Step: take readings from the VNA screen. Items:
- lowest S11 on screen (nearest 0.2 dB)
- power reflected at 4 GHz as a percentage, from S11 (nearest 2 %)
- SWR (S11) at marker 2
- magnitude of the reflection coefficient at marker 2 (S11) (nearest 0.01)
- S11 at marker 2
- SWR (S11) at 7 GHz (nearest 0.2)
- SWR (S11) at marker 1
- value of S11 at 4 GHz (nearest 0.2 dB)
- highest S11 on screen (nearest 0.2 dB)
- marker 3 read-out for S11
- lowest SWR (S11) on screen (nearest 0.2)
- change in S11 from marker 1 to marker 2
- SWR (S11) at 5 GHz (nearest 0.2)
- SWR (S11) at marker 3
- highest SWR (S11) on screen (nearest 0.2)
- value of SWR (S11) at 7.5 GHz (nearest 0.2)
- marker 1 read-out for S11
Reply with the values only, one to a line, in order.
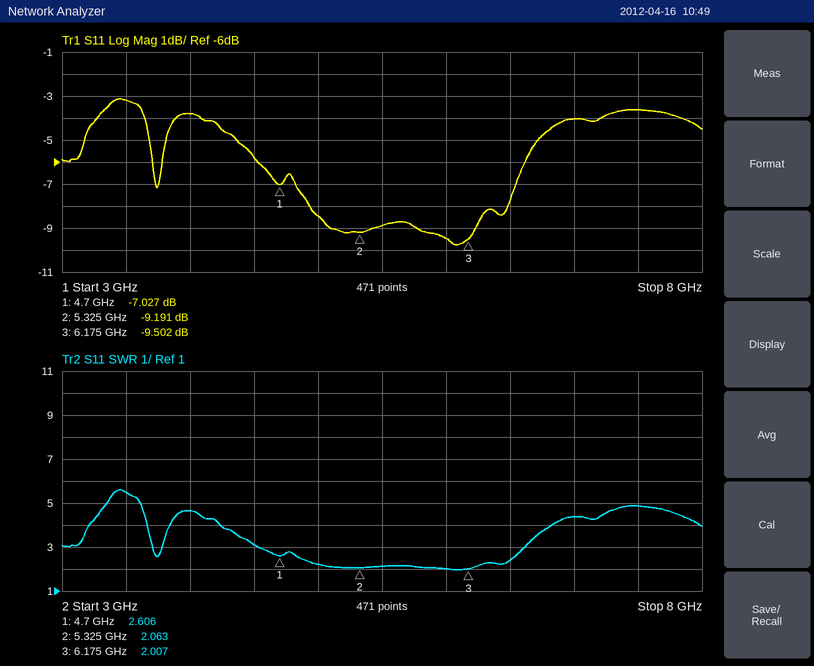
-9.8 dB
42 %
2.063
0.35
-9.191 dB
4.4
2.606
-3.8 dB
-3.2 dB
-9.502 dB
2.0
-2.164 dB
2.2
2.007
5.6
4.8
-7.027 dB
